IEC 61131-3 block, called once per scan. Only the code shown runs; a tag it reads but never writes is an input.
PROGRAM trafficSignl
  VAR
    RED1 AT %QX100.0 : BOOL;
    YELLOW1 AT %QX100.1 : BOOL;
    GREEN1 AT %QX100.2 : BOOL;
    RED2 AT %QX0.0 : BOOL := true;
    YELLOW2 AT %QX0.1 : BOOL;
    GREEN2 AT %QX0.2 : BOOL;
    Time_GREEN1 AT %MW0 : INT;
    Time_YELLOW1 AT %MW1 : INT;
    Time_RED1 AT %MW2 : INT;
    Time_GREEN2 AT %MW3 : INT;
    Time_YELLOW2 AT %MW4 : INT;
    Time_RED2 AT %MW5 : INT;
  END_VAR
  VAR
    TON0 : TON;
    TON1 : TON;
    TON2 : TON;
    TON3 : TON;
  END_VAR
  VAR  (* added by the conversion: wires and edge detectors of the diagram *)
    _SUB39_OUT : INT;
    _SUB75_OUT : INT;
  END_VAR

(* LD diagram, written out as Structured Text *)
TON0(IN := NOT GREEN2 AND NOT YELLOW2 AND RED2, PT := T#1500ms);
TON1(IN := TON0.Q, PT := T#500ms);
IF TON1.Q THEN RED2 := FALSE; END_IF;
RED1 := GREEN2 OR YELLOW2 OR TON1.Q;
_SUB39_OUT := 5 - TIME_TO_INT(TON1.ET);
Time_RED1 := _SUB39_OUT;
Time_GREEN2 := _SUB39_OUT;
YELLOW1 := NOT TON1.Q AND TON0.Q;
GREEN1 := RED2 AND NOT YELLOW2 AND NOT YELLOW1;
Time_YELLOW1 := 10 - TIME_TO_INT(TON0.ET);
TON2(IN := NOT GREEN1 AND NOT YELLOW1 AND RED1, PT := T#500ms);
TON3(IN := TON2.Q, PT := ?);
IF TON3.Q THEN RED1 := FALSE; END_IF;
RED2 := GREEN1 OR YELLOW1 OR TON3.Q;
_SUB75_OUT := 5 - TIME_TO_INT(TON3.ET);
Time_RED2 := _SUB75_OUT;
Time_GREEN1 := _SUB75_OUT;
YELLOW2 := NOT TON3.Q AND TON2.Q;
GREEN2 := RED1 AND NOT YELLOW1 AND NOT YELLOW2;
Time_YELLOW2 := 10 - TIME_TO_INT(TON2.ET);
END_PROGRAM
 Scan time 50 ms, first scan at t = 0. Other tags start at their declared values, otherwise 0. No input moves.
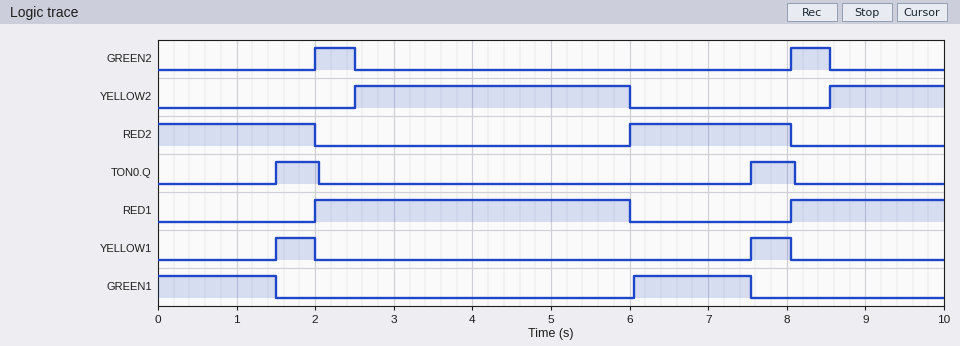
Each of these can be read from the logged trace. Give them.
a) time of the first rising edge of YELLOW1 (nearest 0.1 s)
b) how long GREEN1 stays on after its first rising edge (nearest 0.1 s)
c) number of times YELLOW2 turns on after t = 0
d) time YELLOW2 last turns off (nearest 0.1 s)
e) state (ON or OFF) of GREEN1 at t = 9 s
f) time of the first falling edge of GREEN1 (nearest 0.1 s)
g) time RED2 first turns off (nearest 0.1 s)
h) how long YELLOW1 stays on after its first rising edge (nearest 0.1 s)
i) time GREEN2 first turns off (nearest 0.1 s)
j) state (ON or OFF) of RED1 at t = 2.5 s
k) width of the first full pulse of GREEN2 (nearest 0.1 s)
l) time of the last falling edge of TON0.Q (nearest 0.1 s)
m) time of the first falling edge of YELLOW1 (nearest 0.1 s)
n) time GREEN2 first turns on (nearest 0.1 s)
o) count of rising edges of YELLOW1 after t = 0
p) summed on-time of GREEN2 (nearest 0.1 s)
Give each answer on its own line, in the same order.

1.5 s
1.5 s
2
6.0 s
OFF
1.5 s
2.0 s
0.5 s
2.5 s
ON
0.5 s
8.1 s
2.0 s
2.0 s
2
1.0 s
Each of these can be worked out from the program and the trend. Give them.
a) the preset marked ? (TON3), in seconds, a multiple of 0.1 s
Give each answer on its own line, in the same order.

3.5 s
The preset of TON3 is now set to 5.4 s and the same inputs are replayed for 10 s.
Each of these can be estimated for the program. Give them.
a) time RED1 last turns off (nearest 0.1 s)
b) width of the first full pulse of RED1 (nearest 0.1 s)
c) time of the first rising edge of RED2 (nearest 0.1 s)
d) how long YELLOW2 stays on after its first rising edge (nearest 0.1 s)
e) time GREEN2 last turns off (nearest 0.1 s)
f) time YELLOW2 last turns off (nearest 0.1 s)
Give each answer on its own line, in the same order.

7.9 s
5.9 s
7.9 s
5.4 s
2.5 s
7.9 s
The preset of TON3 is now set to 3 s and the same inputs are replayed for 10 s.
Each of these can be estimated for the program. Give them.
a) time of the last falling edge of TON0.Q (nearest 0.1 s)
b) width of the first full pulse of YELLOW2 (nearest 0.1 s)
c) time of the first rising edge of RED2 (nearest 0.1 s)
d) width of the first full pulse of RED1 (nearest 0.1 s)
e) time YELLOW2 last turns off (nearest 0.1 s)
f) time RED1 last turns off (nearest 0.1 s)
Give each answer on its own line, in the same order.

7.6 s
3.0 s
5.5 s
3.5 s
5.5 s
5.5 s
